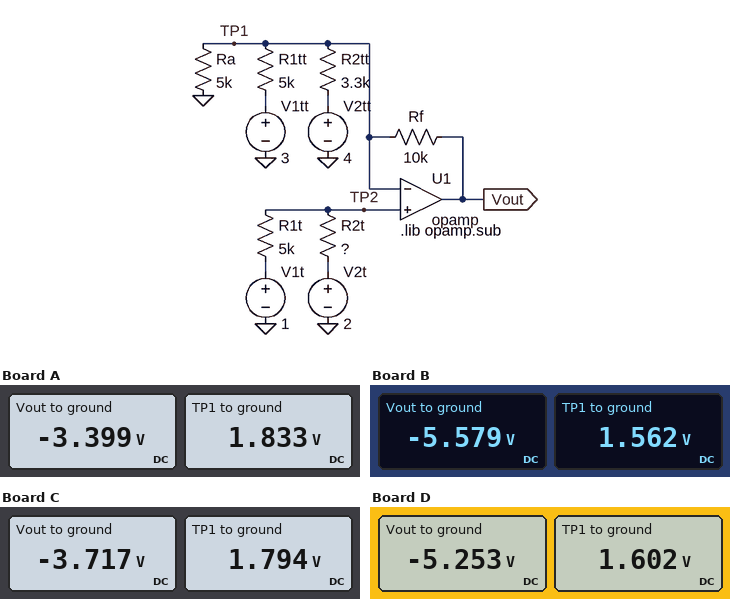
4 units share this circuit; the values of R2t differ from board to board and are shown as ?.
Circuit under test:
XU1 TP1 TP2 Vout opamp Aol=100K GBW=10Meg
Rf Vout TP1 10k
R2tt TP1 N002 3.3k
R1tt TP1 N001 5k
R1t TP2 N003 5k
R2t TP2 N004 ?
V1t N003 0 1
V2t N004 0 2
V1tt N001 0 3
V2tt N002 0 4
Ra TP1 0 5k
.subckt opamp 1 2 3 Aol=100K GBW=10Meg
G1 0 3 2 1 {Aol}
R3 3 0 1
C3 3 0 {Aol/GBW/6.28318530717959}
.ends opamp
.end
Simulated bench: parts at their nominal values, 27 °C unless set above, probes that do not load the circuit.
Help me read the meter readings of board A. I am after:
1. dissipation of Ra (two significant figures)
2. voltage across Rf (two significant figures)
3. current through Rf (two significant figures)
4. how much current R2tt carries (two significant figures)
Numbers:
670 µW
5.2 V
520 µA
660 µA
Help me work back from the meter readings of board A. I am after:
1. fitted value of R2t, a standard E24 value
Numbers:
1 kΩ
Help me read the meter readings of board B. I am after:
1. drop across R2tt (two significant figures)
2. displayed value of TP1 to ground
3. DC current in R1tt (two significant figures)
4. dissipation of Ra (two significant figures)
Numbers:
2.4 V
1.562 V
290 µA
490 µW
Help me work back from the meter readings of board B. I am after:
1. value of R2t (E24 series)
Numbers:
3.9 kΩ
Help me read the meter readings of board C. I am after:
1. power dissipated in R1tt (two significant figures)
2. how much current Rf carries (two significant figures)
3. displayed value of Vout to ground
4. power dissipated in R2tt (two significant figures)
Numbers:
290 µW
550 µA
-3.717 V
1.5 mW
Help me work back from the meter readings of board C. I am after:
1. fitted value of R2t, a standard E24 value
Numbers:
1.3 kΩ
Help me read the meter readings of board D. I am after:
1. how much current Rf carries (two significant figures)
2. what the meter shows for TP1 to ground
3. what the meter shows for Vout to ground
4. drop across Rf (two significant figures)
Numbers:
690 µA
1.602 V
-5.253 V
6.9 V
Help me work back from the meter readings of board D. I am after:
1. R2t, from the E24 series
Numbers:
3.3 kΩ
